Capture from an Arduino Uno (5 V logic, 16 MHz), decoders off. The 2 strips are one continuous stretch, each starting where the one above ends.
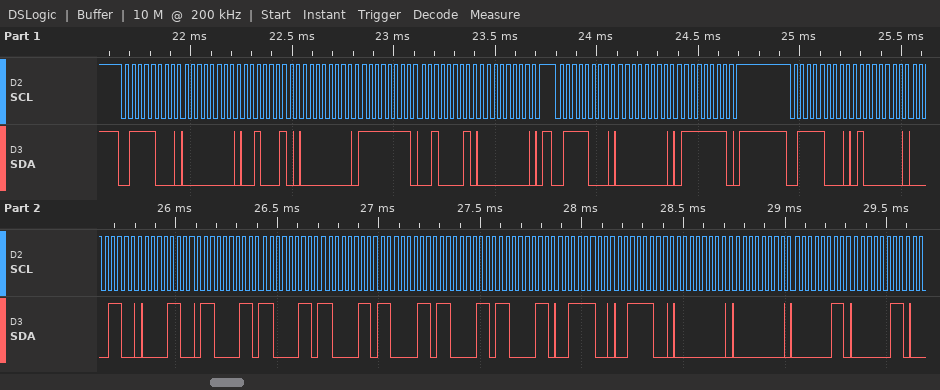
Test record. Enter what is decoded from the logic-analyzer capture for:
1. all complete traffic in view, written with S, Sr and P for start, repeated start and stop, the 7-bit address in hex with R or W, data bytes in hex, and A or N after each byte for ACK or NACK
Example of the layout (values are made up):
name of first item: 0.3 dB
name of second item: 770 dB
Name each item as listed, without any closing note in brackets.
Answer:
all complete traffic in view, written with S, Sr and P for start, repeated start and stop, the 7-bit address in hex with R or W, data bytes in hex, and A or N after each byte for ACK or NACK: S 3CW A 00 A 22 A 00 A FF A 21 A 00 A P S 3CW A 00 A 7F A P S 3CW A 40 A 0C A 0C A C3 A C3 A C3 A C3 A C3 A C3 A 3C A 3C A 00 A 00 A 03 A 03 A
